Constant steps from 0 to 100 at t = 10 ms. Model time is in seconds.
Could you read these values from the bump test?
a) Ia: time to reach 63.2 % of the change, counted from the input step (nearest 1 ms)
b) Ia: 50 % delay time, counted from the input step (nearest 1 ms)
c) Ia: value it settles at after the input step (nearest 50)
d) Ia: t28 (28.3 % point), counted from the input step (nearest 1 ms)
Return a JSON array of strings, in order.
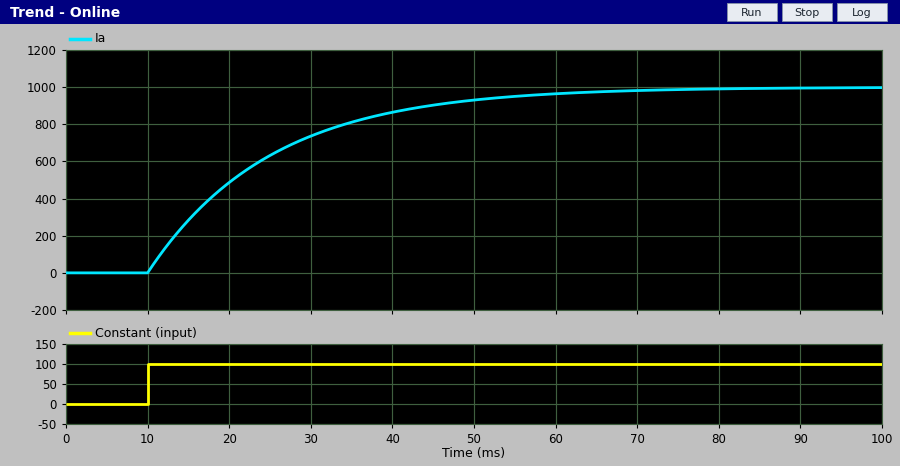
["15 ms", "10 ms", "1000", "5 ms"]
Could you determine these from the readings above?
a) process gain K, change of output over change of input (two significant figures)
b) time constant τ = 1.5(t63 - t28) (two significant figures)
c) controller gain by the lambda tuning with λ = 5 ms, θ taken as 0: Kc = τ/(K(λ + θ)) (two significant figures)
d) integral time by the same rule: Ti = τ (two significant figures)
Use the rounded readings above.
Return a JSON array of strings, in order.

["10", "15 ms", "0.30", "15 ms"]
